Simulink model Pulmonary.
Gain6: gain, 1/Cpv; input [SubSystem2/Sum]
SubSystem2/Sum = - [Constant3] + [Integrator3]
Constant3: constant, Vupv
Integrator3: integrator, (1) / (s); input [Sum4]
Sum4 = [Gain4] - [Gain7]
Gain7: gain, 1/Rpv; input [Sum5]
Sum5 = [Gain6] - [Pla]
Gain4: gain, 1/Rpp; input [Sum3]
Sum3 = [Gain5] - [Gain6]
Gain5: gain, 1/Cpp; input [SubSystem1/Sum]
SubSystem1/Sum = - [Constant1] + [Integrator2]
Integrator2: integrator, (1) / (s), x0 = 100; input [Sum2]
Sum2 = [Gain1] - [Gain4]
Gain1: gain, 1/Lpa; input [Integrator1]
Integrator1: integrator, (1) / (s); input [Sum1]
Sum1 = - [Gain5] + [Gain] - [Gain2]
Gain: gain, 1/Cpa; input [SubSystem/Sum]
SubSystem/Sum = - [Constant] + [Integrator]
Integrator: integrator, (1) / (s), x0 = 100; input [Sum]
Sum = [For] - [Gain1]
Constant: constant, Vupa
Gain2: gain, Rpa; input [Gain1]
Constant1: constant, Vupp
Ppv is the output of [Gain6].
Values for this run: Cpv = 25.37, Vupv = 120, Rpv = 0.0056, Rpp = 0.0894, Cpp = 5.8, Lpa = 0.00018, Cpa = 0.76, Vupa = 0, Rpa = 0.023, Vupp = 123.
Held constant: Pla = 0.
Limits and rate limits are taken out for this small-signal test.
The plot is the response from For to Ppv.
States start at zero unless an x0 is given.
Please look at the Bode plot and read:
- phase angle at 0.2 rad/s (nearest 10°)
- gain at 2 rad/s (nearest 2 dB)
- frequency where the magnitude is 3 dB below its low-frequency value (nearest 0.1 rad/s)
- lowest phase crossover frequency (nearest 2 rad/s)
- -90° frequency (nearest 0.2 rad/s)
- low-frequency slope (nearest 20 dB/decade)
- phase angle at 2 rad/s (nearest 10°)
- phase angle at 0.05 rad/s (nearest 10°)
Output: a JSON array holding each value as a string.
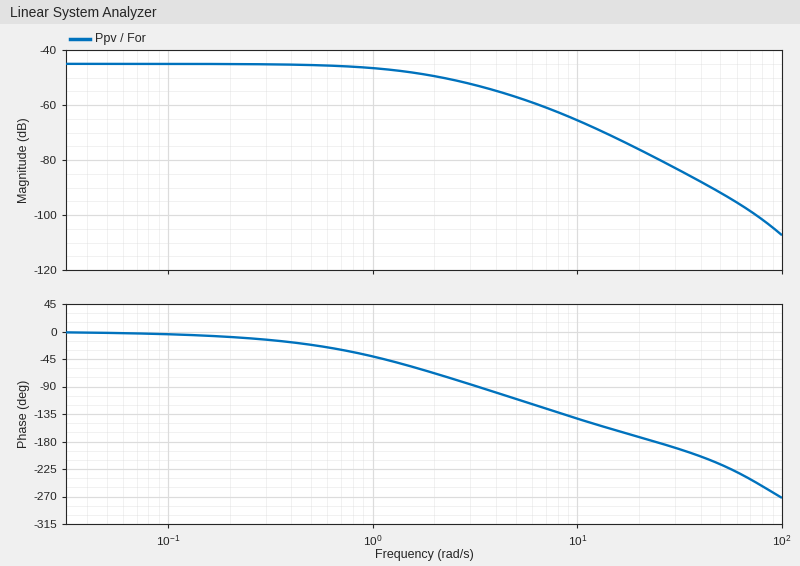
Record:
["-10°", "-50 dB", "1.5 rad/s", "24 rad/s", "3.2 rad/s", "0 dB/decade", "-70°", "0°"]
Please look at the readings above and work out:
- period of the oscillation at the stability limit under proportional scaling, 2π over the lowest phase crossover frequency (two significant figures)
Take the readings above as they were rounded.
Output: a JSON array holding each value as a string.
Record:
["0.26 s"]
